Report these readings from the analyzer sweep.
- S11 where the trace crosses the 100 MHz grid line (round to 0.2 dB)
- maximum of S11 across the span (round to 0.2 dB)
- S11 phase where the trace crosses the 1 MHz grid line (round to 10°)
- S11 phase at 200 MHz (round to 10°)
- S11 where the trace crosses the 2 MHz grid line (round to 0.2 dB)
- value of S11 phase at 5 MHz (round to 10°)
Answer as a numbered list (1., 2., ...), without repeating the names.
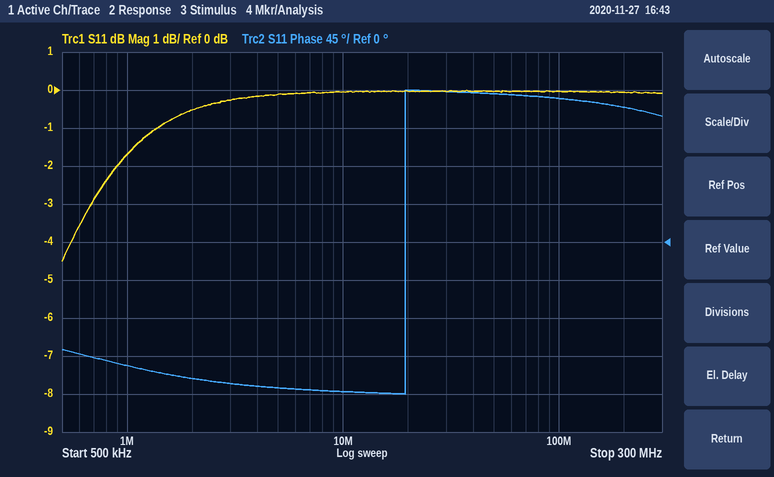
1. 0.0 dB
2. 0.0 dB
3. -150°
4. 160°
5. -0.6 dB
6. -170°
